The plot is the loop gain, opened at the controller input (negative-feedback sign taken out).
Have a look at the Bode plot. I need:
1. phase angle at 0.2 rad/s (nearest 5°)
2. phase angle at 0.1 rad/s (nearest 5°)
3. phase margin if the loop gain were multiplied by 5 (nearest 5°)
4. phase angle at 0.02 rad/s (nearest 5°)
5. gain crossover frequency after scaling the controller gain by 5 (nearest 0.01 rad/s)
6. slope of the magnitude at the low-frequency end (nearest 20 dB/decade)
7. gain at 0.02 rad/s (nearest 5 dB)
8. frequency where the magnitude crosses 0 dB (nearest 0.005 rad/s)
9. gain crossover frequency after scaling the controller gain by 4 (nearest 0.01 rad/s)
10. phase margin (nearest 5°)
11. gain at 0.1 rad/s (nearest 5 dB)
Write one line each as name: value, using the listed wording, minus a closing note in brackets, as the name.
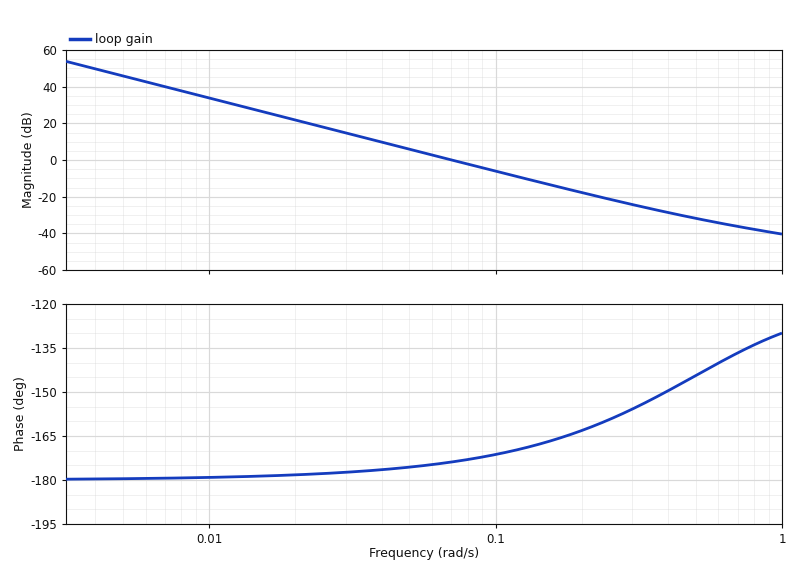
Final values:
phase angle at 0.2 rad/s: -165°
phase angle at 0.1 rad/s: -170°
phase margin if the loop gain were multiplied by 5: 15°
phase angle at 0.02 rad/s: -180°
gain crossover frequency after scaling the controller gain by 5: 0.16 rad/s
slope of the magnitude at the low-frequency end: -40 dB/decade
gain at 0.02 rad/s: 20 dB
frequency where the magnitude crosses 0 dB: 0.070 rad/s
gain crossover frequency after scaling the controller gain by 4: 0.14 rad/s
phase margin: 5°
gain at 0.1 rad/s: -5 dB
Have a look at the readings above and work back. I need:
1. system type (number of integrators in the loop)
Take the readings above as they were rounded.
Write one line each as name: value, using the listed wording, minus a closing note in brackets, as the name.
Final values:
system type: 2
